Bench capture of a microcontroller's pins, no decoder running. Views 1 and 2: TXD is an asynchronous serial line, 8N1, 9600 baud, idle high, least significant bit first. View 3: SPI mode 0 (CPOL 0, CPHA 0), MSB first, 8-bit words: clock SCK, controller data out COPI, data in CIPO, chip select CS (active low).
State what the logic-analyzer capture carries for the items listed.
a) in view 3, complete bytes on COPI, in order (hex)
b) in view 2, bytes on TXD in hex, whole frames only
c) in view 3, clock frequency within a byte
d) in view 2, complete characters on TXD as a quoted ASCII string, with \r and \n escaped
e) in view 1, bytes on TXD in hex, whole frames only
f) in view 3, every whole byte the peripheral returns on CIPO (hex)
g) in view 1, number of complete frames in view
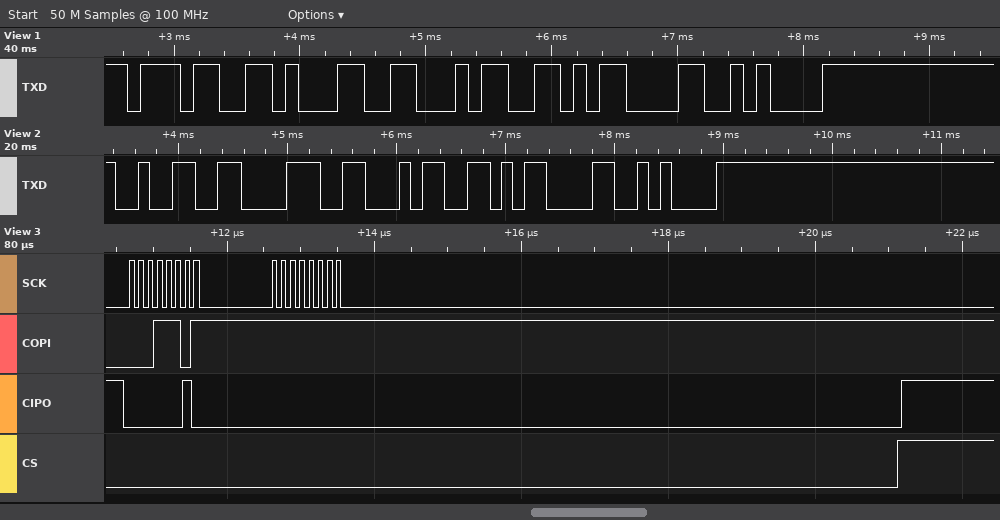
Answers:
1D FF
32 38 34 0D 0A
8 MHz
"284\r\n"
37 31 34 0D 0A
02 00
5
